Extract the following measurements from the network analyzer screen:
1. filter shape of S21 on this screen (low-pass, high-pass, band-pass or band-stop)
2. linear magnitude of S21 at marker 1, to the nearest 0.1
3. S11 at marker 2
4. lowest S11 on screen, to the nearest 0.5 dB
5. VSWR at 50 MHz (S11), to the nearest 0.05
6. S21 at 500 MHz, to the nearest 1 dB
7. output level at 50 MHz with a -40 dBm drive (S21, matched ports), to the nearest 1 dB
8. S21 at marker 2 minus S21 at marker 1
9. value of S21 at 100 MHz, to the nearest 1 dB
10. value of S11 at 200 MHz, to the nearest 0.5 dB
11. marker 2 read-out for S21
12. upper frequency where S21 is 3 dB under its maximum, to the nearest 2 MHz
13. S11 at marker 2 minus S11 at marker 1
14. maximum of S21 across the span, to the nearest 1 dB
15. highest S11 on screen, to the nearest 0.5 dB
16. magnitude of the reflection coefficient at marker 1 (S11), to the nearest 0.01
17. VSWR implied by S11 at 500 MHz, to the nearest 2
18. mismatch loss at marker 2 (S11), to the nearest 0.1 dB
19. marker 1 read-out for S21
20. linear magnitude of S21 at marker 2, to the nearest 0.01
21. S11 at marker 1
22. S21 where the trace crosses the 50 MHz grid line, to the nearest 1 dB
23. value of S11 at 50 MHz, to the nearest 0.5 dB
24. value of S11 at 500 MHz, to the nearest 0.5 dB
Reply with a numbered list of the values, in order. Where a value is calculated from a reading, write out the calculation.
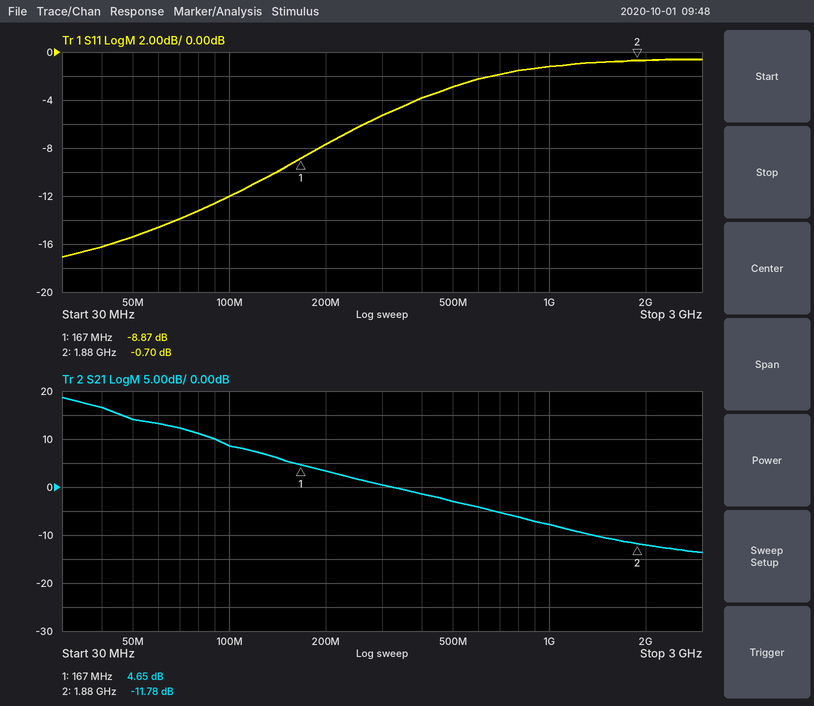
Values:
1. low-pass
2. 10^(4.65/20) ≈ 1.7
3. -0.70 dB
4. -17.0 dB
5. |Γ| = 10^(-15.5/20) = 0.1679; VSWR = (1 + 0.1679)/(1 − 0.1679) ≈ 1.40
6. -3 dB
7. -40 dBm + (14 dB) = -26 dBm
8. -11.78 − (4.65) = -16.43 dB
9. 9 dB
10. -7.5 dB
11. -11.78 dB
12. 44 MHz
13. -0.7 − (-8.87) = 8.17 dB
14. 19 dB
15. -0.5 dB
16. 10^(-8.87/20) ≈ 0.36
17. |Γ| = 10^(-3/20) = 0.7079; VSWR = (1 + 0.7079)/(1 − 0.7079) ≈ 6
18. −10 log10(1 − 10^(-0.7/10)) ≈ 8.3 dB
19. 4.65 dB
20. 10^(-11.78/20) ≈ 0.26
21. -8.87 dB
22. 14 dB
23. -15.5 dB
24. -3.0 dB
